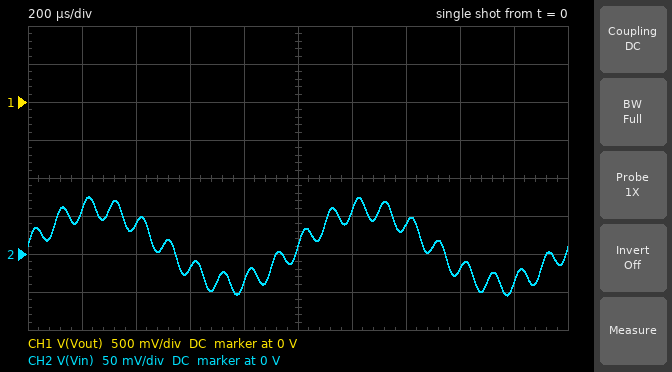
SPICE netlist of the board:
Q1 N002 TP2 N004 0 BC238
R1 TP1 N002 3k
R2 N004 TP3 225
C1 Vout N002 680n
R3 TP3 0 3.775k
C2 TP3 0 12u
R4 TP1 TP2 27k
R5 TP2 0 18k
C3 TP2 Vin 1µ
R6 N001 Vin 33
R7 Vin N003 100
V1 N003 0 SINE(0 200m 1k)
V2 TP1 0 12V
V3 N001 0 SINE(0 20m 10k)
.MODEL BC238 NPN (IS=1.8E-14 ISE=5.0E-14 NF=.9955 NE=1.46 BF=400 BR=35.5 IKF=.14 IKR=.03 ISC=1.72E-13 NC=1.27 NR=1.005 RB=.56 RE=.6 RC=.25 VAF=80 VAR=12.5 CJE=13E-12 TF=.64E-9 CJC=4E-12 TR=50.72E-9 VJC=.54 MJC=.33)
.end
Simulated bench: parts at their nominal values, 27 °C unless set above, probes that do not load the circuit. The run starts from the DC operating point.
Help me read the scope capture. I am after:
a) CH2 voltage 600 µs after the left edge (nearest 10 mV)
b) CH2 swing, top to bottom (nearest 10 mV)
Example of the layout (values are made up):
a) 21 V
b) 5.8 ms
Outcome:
a) -20 mV
b) 130 mV
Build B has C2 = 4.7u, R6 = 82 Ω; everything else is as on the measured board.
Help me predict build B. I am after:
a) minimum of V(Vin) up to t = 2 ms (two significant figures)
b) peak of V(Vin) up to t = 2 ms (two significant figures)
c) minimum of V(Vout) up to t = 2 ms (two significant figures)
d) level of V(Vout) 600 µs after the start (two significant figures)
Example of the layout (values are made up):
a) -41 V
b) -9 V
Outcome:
a) -83 mV
b) 120 mV
c) 9.9 V
d) 12 V
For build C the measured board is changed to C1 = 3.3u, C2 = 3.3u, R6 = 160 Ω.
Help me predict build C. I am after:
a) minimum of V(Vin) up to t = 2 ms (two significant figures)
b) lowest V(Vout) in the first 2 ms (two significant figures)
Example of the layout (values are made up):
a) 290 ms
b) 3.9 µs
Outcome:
a) -110 mV
b) 10 V
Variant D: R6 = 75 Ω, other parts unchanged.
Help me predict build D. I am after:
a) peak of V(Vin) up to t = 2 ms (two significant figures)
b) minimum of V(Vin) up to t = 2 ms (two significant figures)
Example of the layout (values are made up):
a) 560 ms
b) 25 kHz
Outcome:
a) 110 mV
b) -80 mV
